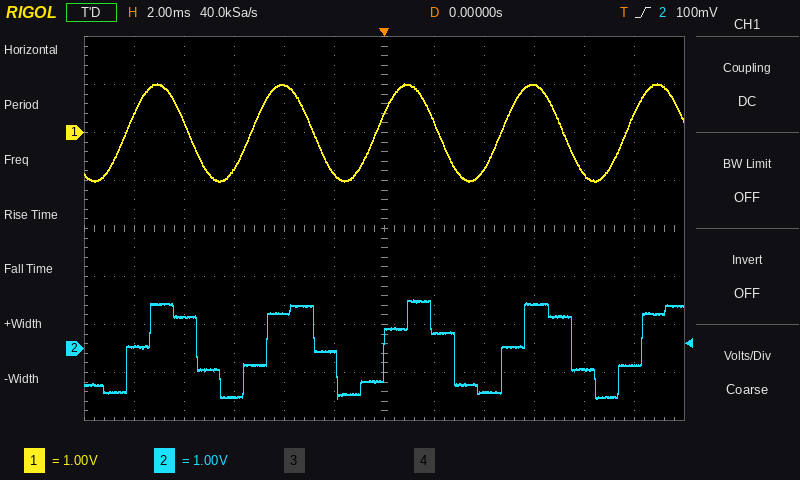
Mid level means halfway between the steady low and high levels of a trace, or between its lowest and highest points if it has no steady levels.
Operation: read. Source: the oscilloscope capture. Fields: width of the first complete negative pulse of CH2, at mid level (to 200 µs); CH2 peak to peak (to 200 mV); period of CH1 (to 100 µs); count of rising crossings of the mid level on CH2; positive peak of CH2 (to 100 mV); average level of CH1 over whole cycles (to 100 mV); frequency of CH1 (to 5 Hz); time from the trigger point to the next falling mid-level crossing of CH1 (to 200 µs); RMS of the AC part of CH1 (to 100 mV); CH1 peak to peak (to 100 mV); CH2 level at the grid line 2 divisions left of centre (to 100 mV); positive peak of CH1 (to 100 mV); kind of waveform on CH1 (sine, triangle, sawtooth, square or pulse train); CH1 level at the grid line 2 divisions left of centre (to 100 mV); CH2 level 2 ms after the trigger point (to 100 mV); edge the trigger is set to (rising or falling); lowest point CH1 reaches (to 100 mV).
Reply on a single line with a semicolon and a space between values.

2.8 ms; 2.0 V; 5.0 ms; 5; 1.0 V; 0.0 V; 200 Hz; 2.2 ms; 700 mV; 2.0 V; 700 mV; 1.0 V; sine; 1.0 V; 400 mV; rising; -1.0 V
